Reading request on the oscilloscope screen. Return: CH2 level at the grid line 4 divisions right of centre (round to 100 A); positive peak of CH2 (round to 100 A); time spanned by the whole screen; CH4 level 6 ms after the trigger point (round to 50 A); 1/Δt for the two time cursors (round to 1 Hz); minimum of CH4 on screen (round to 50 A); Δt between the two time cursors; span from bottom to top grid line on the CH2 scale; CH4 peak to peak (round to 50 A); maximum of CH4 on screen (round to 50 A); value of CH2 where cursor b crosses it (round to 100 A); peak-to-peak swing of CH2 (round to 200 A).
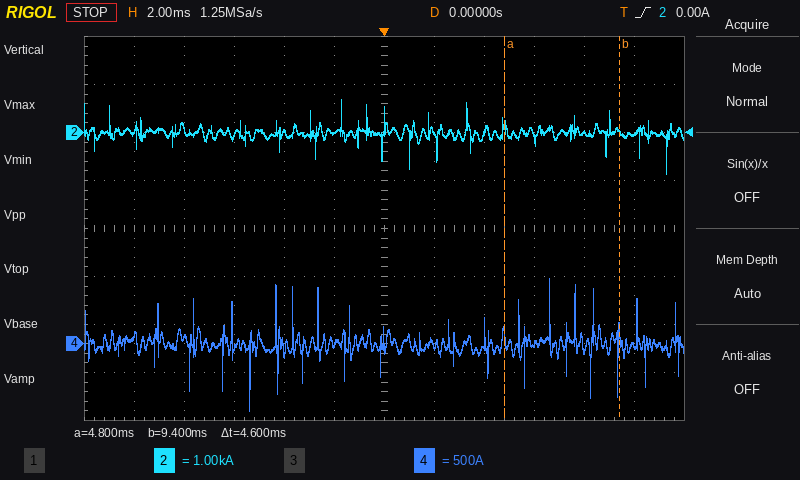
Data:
0.0 kA
700 A
24 ms
0 A
217 Hz
-700 A
4.6 ms
8 kA
1.40 kA
700 A
0.0 kA
1.6 kA
